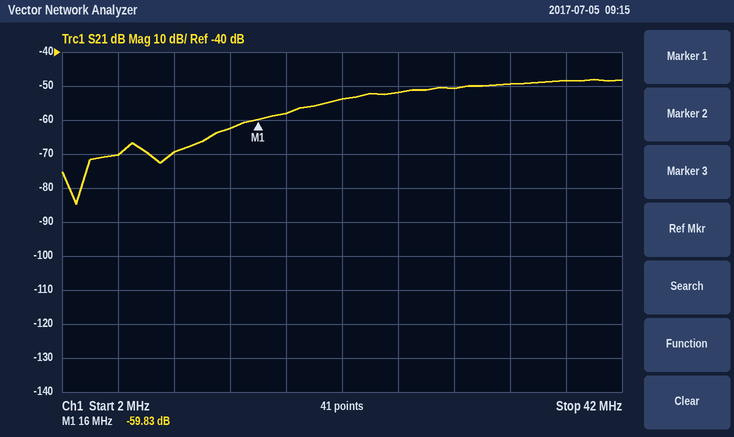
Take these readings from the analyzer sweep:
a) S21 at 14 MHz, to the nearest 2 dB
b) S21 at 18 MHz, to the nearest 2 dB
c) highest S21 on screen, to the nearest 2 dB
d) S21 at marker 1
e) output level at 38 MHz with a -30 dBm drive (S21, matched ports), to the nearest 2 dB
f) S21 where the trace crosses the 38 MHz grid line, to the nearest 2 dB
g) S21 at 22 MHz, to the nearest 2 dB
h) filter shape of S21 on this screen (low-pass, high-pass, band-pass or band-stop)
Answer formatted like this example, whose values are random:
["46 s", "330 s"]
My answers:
["-62 dB", "-58 dB", "-48 dB", "-59.83 dB", "-78 dBm", "-48 dB", "-54 dB", "high-pass"]
